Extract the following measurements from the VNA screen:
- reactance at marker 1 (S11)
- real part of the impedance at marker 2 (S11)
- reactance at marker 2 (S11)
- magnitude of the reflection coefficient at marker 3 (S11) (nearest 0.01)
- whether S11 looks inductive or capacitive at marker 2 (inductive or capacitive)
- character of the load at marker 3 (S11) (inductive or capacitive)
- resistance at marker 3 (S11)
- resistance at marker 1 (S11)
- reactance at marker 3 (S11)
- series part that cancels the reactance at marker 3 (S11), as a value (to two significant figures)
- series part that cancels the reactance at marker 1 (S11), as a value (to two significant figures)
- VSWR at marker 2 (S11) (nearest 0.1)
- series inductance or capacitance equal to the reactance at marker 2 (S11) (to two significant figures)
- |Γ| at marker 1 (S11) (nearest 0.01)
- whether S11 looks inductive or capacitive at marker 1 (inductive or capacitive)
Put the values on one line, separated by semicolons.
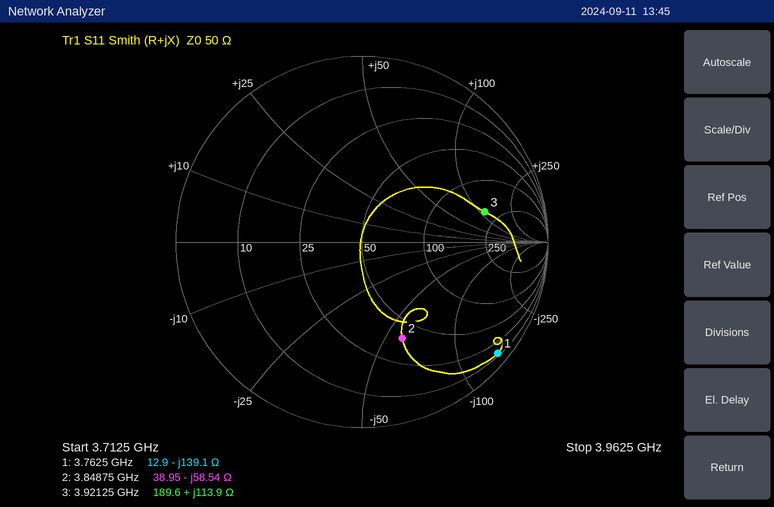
-139.1 Ω; 38.95 Ω; -58.54 Ω; 0.68; capacitive; inductive; 189.6 Ω; 12.9 Ω; +113.9 Ω; 360 fF; 5.9 nH; 3.5; 710 fF; 0.94; capacitive
